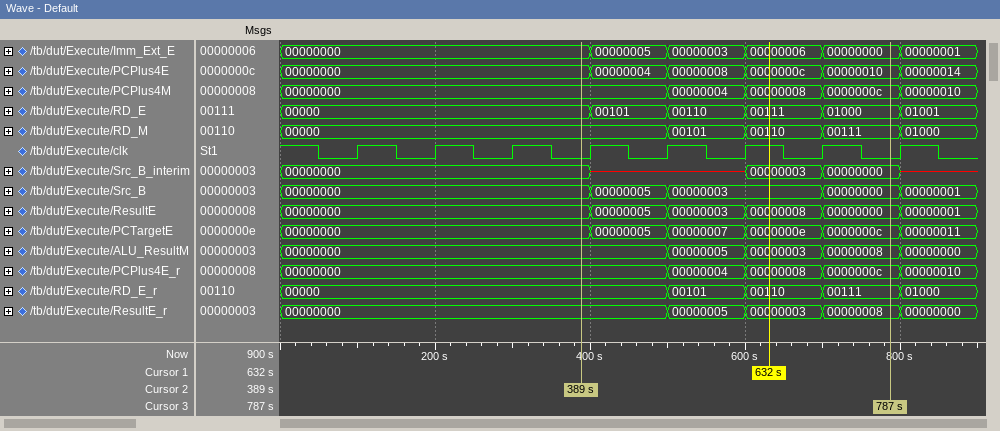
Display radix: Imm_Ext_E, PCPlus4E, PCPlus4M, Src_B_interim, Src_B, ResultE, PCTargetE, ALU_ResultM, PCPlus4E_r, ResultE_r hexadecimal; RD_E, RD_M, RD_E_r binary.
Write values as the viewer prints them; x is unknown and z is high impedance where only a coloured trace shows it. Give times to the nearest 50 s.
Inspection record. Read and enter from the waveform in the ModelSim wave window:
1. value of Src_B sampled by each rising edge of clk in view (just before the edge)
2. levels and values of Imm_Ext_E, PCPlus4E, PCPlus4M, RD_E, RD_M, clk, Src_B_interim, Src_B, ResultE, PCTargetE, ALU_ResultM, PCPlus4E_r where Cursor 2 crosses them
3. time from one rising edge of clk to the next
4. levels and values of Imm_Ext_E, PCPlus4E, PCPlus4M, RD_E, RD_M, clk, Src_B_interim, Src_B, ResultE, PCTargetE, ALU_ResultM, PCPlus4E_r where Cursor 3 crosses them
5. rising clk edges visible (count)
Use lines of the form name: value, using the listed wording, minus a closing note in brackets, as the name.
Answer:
value of Src_B sampled by each rising edge of clk in view: 00000000, 00000000, 00000000, 00000000, 00000005, 00000003, 00000003, 00000000
levels and values of Imm_Ext_E, PCPlus4E, PCPlus4M, RD_E, RD_M, clk, Src_B_interim, Src_B, ResultE, PCTargetE, ALU_ResultM, PCPlus4E_r where Cursor 2 crosses them: Imm_Ext_E=00000000, PCPlus4E=00000000, PCPlus4M=00000000, RD_E=00000, RD_M=00000, clk=0, Src_B_interim=00000000, Src_B=00000000, ResultE=00000000, PCTargetE=00000000, ALU_ResultM=00000000, PCPlus4E_r=00000000
time from one rising edge of clk to the next: 100 s
levels and values of Imm_Ext_E, PCPlus4E, PCPlus4M, RD_E, RD_M, clk, Src_B_interim, Src_B, ResultE, PCTargetE, ALU_ResultM, PCPlus4E_r where Cursor 3 crosses them: Imm_Ext_E=00000000, PCPlus4E=00000010, PCPlus4M=0000000c, RD_E=01000, RD_M=00111, clk=0, Src_B_interim=00000000, Src_B=00000000, ResultE=00000000, PCTargetE=0000000c, ALU_ResultM=00000008, PCPlus4E_r=0000000c
rising clk edges visible: 8
